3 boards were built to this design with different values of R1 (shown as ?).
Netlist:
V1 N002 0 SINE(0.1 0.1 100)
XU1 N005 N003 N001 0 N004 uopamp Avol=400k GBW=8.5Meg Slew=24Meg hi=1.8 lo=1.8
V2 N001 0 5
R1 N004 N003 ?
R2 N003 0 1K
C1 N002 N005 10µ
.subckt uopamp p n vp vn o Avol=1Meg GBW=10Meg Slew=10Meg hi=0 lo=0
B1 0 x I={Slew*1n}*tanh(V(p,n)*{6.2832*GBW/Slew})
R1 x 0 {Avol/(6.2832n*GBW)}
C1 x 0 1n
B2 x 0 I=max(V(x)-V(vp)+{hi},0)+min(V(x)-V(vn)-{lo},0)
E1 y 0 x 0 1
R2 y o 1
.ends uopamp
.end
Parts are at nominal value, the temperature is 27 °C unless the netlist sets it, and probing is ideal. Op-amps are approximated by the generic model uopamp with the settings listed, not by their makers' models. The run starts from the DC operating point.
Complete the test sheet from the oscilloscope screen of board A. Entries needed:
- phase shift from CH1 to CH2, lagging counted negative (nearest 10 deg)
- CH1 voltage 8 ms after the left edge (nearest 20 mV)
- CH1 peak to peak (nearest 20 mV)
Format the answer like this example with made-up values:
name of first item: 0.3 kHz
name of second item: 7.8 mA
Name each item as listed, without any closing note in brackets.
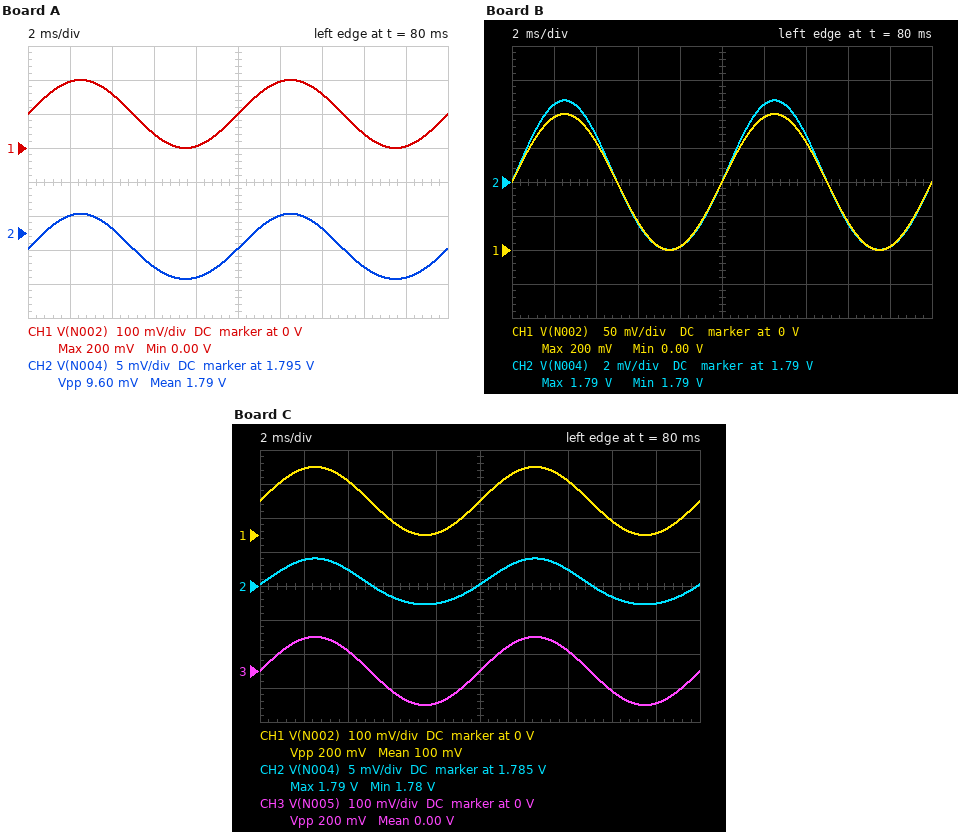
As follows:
phase shift from CH1 to CH2, lagging counted negative: 0 deg
CH1 voltage 8 ms after the left edge: 0 V
CH1 peak to peak: 200 mV
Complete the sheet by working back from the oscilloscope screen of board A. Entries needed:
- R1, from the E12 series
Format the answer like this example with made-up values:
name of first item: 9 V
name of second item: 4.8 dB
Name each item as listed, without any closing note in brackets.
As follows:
R1, from the E12 series: 12 kΩ
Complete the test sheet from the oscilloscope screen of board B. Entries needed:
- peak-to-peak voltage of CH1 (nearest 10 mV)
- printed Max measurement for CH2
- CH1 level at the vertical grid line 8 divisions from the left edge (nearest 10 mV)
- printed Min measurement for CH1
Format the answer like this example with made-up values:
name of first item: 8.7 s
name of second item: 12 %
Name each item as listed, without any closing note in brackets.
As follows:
peak-to-peak voltage of CH1: 200 mV
printed Max measurement for CH2: 1.79 V
CH1 level at the vertical grid line 8 divisions from the left edge: 40 mV
printed Min measurement for CH1: 0.00 V
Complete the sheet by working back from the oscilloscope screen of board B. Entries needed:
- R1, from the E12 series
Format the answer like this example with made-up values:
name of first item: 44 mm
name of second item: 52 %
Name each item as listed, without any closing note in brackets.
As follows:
R1, from the E12 series: 8.2 kΩ
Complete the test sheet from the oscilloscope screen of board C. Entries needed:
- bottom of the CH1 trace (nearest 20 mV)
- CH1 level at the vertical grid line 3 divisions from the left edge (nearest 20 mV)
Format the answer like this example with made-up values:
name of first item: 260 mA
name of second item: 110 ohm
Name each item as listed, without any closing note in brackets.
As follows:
bottom of the CH1 trace: 0 V
CH1 level at the vertical grid line 3 divisions from the left edge: 40 mV
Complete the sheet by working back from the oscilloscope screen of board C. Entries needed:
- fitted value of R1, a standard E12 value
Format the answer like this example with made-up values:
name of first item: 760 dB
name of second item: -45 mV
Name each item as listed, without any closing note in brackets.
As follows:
fitted value of R1, a standard E12 value: 4.7 kΩ
